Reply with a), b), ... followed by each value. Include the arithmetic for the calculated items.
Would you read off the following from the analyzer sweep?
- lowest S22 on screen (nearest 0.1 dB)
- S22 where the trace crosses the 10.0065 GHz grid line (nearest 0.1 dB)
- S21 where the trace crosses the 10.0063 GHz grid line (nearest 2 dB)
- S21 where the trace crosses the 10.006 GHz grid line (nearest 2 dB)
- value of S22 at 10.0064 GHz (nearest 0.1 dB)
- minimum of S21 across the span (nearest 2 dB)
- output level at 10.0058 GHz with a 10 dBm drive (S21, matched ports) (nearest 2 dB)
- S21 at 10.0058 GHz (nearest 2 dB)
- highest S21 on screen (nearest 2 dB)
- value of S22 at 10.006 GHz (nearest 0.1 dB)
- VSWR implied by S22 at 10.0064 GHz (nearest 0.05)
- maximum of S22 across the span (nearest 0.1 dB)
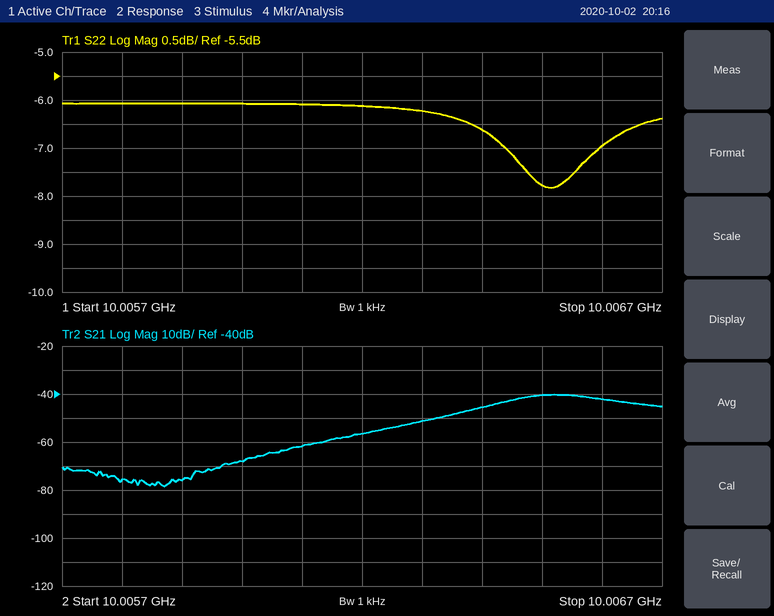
a) -7.8 dB
b) -7.8 dB
c) -52 dB
d) -68 dB
e) -6.6 dB
f) -78 dB
g) 10 dBm + (-76 dB) = -66 dBm
h) -76 dB
i) -40 dB
j) -6.1 dB
k) |Γ| = 10^(-6.6/20) = 0.4677; VSWR = (1 + 0.4677)/(1 − 0.4677) ≈ 2.76, so 2.75 to the nearest 0.05
l) -6.1 dB
